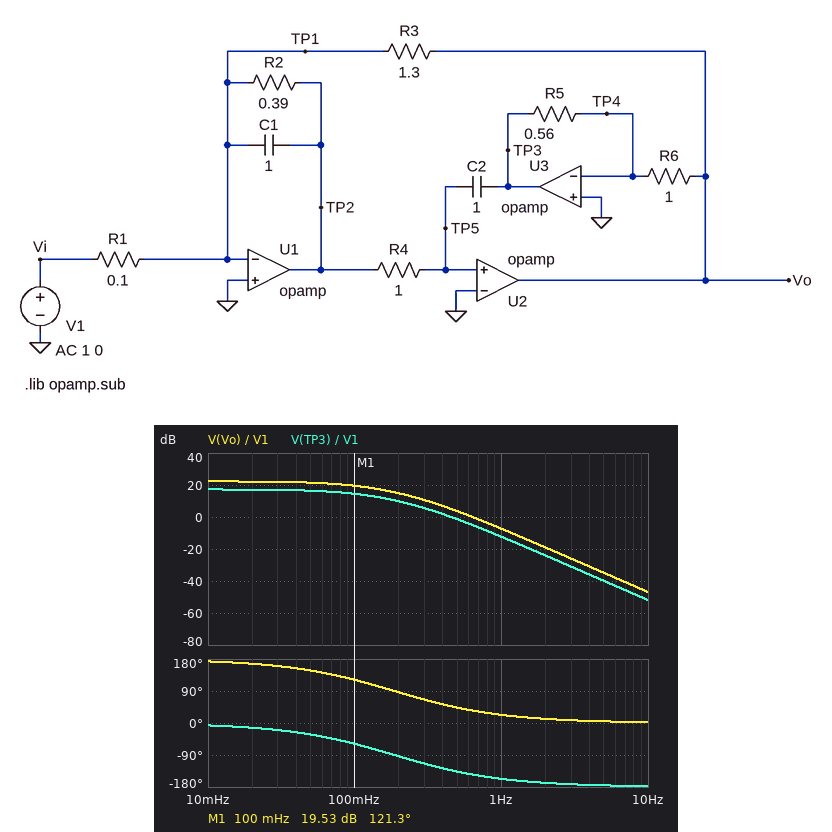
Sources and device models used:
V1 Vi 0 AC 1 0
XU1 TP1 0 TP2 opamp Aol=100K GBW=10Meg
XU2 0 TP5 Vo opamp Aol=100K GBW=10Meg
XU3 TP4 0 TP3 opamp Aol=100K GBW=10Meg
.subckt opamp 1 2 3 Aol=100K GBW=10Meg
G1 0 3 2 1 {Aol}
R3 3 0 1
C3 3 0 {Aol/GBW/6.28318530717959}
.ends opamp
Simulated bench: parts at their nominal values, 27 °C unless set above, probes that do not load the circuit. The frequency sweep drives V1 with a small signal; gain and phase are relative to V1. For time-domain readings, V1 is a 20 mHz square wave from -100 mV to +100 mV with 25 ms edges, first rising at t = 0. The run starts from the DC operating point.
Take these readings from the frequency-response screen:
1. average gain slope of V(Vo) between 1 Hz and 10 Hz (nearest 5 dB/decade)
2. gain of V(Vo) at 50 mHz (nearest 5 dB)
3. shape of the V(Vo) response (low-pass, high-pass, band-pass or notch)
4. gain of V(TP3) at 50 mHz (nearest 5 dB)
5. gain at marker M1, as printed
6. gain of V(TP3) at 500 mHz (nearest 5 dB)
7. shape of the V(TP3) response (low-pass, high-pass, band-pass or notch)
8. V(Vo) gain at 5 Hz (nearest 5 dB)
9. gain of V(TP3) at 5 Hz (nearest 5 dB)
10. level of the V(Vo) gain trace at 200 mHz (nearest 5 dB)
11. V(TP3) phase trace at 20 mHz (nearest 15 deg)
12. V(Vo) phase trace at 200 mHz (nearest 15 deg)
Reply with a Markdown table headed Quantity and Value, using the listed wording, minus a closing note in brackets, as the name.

| Quantity | Value |
|---|---|
| average gain slope of V(Vo) between 1 Hz and 10 Hz | -40 dB/decade |
| gain of V(Vo) at 50 mHz | 20 dB |
| shape of the V(Vo) response | low-pass |
| gain of V(TP3) at 50 mHz | 15 dB |
| gain at marker M1, as printed | 19.53 dB |
| gain of V(TP3) at 500 mHz | 0 dB |
| shape of the V(TP3) response | low-pass |
| V(Vo) gain at 5 Hz | -35 dB |
| gain of V(TP3) at 5 Hz | -40 dB |
| level of the V(Vo) gain trace at 200 mHz | 15 dB |
| V(TP3) phase trace at 20 mHz | -15 deg |
| V(Vo) phase trace at 200 mHz | 90 deg |
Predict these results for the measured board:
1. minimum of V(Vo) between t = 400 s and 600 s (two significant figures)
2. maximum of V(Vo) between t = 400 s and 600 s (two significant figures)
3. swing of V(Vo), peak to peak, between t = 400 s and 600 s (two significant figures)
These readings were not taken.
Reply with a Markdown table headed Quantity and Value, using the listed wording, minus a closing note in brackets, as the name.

| Quantity | Value |
|---|---|
| minimum of V(Vo) between t = 400 s and 600 s | -1.3 V |
| maximum of V(Vo) between t = 400 s and 600 s | 1.3 V |
| swing of V(Vo), peak to peak, between t = 400 s and 600 s | 2.6 V |
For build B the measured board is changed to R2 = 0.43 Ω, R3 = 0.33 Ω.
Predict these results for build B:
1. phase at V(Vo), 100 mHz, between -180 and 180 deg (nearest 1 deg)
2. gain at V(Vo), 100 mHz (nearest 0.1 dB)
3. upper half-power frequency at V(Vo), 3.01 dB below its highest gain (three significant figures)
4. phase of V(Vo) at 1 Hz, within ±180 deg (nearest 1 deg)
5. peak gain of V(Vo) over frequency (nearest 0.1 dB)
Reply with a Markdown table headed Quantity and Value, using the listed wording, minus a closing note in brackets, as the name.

| Quantity | Value |
|---|---|
| phase at V(Vo), 100 mHz, between -180 and 180 deg | 164 deg |
| gain at V(Vo), 100 mHz | 10.7 dB |
| upper half-power frequency at V(Vo), 3.01 dB below its highest gain | 433 mHz |
| phase of V(Vo) at 1 Hz, within ±180 deg | 23 deg |
| peak gain of V(Vo) over frequency | 11.6 dB |
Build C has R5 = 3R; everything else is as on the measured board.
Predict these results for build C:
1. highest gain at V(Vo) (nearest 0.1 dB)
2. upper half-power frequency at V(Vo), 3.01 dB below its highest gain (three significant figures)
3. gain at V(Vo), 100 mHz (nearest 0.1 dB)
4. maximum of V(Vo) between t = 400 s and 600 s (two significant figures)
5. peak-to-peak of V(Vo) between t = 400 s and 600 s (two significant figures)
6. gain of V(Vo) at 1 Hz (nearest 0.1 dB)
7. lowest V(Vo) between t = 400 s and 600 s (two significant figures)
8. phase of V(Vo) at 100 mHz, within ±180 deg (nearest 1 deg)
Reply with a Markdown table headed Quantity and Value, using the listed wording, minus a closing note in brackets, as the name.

| Quantity | Value |
|---|---|
| highest gain at V(Vo) | 22.3 dB |
| upper half-power frequency at V(Vo), 3.01 dB below its highest gain | 16.6 mHz |
| gain at V(Vo), 100 mHz | 6.3 dB |
| maximum of V(Vo) between t = 400 s and 600 s | 1.1 V |
| peak-to-peak of V(Vo) between t = 400 s and 600 s | 2.2 V |
| gain of V(Vo) at 1 Hz | -22.1 dB |
| lowest V(Vo) between t = 400 s and 600 s | -1.1 V |
| phase of V(Vo) at 100 mHz, within ±180 deg | 85 deg |
